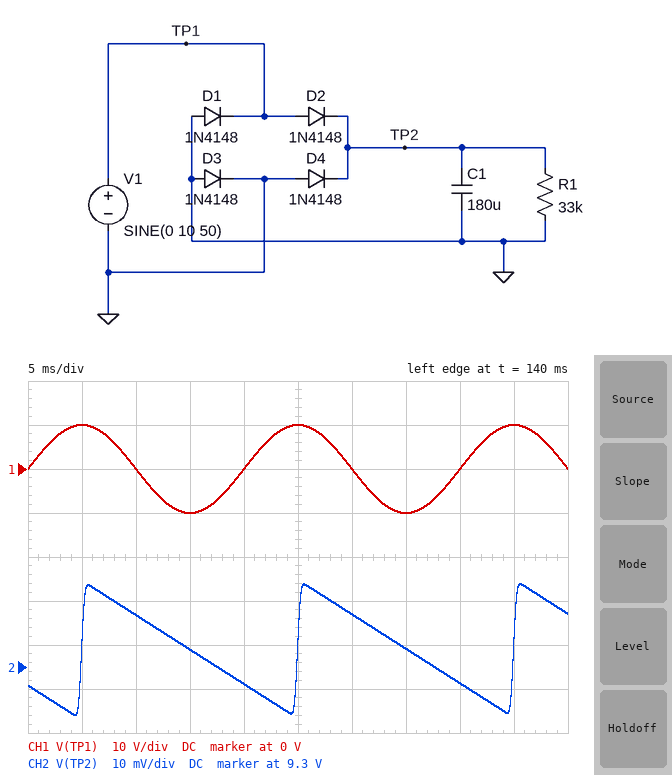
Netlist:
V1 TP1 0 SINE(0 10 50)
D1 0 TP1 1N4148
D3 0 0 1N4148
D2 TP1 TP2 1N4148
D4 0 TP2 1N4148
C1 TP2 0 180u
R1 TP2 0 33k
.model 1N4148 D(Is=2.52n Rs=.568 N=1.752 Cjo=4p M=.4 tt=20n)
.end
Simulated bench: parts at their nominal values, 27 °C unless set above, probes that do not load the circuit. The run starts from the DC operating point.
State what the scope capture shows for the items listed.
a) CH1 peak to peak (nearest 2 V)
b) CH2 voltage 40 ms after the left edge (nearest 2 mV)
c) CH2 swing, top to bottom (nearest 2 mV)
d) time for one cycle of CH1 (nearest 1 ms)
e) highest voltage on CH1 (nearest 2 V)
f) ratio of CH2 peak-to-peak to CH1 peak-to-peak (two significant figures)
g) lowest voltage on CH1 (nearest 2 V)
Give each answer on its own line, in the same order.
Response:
20 V
9.296 V
30 mV
20 ms
10 V
0.0015
-10 V
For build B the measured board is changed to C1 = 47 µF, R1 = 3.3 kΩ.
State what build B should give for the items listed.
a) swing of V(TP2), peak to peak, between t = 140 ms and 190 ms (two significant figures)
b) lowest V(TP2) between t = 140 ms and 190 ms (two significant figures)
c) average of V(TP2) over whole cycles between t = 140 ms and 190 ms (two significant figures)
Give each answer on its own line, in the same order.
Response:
1.0 V
8.3 V
8.8 V
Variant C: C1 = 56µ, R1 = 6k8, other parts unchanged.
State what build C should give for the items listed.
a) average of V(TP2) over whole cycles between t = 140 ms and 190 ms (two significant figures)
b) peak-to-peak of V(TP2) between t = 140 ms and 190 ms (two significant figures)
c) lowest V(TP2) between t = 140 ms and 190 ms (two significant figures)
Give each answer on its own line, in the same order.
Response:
9.1 V
440 mV
8.9 V
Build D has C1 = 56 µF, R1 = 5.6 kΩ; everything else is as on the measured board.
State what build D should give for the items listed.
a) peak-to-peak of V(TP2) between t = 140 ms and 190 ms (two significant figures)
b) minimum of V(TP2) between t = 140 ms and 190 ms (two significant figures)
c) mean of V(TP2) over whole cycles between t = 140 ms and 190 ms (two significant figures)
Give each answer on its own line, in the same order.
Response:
530 mV
8.8 V
9.1 V
